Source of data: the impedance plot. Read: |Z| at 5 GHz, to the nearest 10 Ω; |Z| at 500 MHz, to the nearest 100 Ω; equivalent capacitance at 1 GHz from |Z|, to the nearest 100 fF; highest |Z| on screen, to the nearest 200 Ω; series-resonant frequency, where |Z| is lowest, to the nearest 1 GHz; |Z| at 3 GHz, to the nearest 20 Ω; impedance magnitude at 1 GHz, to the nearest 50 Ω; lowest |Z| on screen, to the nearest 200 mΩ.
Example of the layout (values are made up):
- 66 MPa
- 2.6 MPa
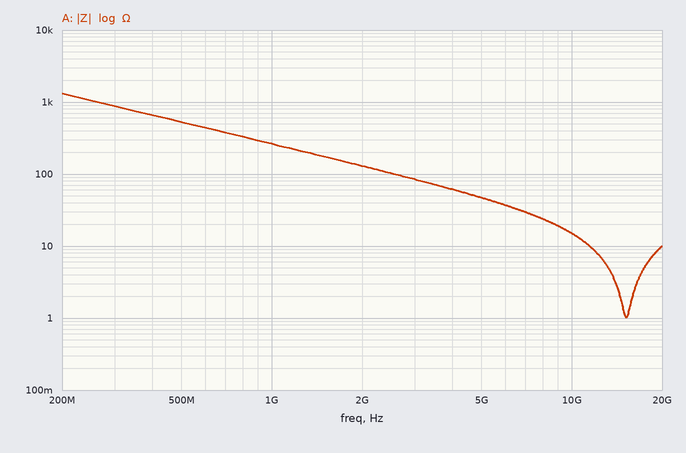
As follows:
- 50 Ω
- 500 Ω
- 600 fF
- 1.4 kΩ
- 15 GHz
- 80 Ω
- 250 Ω
- 1.0 Ω
